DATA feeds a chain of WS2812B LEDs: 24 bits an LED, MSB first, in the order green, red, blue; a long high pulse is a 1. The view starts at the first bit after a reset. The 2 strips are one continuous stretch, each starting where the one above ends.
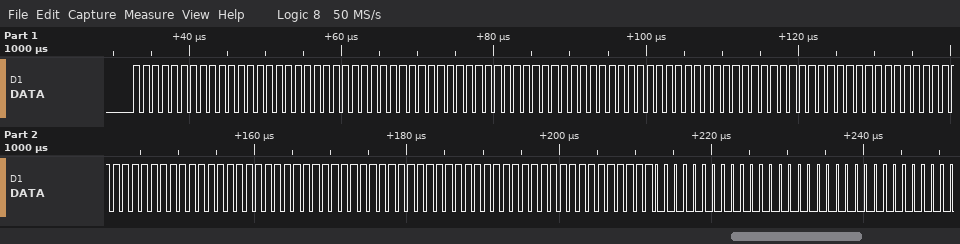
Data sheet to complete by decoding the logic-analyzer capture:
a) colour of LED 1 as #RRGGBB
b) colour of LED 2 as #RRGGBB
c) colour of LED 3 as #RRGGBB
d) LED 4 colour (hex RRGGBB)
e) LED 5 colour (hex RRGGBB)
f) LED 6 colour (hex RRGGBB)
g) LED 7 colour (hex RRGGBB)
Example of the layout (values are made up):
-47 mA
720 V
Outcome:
#FFFFFF
#FFFFFF
#FFFFFF
#FFFFFF
#FFFFFF
#FFFFFF
#000000
